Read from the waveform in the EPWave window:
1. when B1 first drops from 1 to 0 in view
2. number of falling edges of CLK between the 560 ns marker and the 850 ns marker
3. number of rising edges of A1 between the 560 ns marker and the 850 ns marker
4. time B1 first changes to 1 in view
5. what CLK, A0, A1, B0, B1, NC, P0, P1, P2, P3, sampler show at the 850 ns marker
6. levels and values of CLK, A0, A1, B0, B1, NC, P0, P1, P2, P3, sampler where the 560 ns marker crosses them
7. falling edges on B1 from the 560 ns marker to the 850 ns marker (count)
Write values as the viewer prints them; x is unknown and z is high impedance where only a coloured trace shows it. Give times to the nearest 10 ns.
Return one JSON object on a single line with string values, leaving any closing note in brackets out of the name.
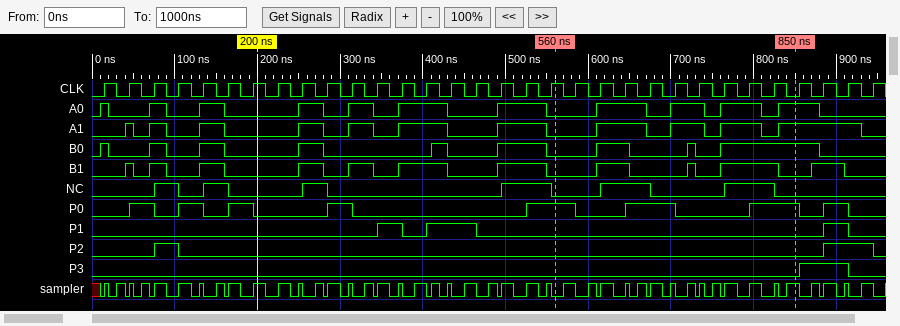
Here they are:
{"when B1 first drops from 1 to 0 in view": "50 ns", "number of falling edges of CLK between the 560 ns marker and the 850 ns marker": "10", "number of rising edges of A1 between the 560 ns marker and the 850 ns marker": "4", "time B1 first changes to 1 in view": "40 ns", "what CLK, A0, A1, B0, B1, NC, P0, P1, P2, P3, sampler show at the 850 ns marker": "CLK=0, A0=1, A1=1, B0=1, B1=0, NC=0, P0=1, P1=0, P2=0, P3=0, sampler=1", "levels and values of CLK, A0, A1, B0, B1, NC, P0, P1, P2, P3, sampler where the 560 ns marker crosses them": "CLK=1, A0=0, A1=0, B0=0, B1=0, NC=0, P0=1, P1=0, P2=0, P3=0, sampler=0", "falling edges on B1 from the 560 ns marker to the 850 ns marker": "3"}
